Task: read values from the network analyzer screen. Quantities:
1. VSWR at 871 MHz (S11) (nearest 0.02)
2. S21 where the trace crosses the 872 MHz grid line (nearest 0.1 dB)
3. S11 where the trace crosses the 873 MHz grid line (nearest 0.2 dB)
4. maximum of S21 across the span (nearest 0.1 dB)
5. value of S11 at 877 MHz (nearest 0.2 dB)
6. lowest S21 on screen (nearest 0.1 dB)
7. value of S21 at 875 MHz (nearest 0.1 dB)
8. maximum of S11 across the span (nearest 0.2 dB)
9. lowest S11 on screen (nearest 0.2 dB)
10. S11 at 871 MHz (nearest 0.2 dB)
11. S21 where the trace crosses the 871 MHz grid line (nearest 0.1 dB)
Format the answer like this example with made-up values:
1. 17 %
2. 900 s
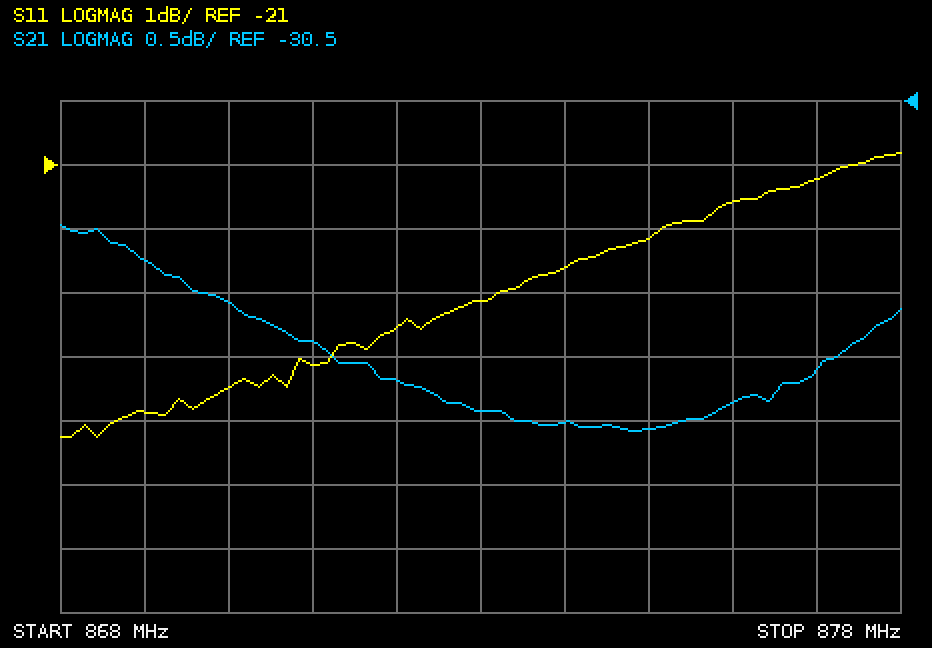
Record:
1. 1.14
2. -32.7 dB
3. -23.2 dB
4. -31.5 dB
5. -21.2 dB
6. -33.1 dB
7. -33.1 dB
8. -20.8 dB
9. -25.2 dB
10. -24.2 dB
11. -32.4 dB
